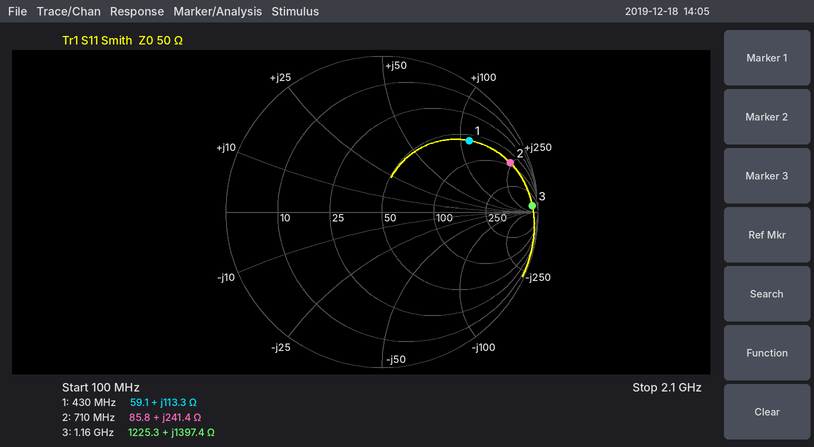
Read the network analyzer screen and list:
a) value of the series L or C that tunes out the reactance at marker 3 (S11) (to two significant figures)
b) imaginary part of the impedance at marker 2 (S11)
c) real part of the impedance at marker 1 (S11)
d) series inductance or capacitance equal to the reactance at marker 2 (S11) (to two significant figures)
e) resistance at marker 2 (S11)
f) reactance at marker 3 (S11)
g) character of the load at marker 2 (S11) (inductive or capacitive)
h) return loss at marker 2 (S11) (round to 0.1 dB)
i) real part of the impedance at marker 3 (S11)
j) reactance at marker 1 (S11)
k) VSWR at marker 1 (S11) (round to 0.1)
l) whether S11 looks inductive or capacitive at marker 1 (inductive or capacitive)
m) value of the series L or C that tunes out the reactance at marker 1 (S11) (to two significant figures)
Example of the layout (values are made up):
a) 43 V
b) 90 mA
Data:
a) 98 fF
b) +241.4 Ω
c) 59.1 Ω
d) 54 nH
e) 85.8 Ω
f) +1397.4 Ω
g) inductive
h) 1.1 dB
i) 1225.3 Ω
j) +113.3 Ω
k) 6.2
l) inductive
m) 3.3 pF
